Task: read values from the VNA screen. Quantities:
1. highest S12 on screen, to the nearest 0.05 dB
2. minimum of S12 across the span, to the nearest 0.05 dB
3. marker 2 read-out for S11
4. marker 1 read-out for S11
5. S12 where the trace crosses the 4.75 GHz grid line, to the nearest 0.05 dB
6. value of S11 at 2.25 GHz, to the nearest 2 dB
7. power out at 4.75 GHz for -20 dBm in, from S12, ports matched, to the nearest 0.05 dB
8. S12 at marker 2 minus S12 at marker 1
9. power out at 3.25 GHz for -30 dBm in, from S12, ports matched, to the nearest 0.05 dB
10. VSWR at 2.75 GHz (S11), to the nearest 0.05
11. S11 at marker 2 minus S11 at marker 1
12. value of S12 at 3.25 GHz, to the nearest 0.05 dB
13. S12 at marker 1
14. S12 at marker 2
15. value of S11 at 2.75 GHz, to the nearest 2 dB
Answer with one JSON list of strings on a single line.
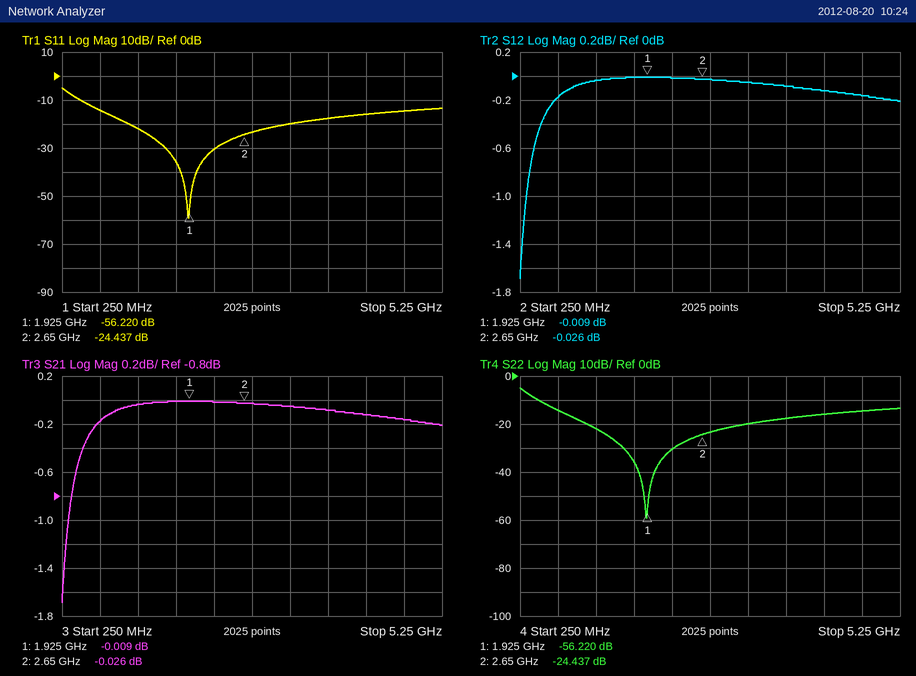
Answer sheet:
["0.00 dB", "-1.70 dB", "-24.437 dB", "-56.220 dB", "-0.15 dB", "-30 dB", "-20.15 dBm", "-0.017 dB", "-30.05 dBm", "1.15", "31.783 dB", "-0.05 dB", "-0.009 dB", "-0.026 dB", "-24 dB"]
